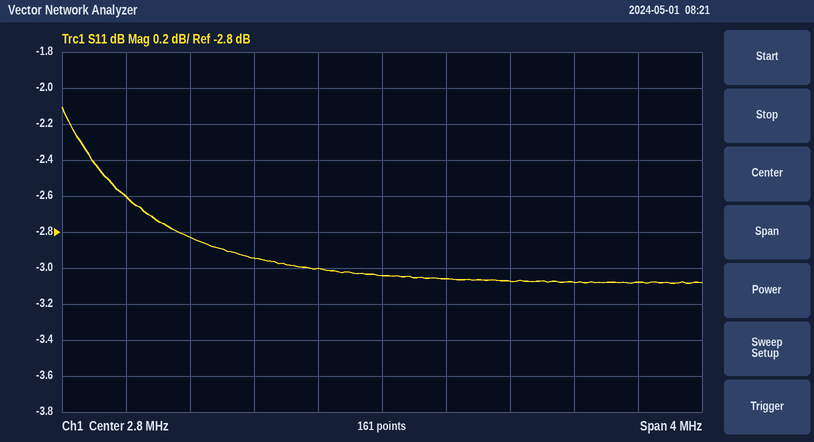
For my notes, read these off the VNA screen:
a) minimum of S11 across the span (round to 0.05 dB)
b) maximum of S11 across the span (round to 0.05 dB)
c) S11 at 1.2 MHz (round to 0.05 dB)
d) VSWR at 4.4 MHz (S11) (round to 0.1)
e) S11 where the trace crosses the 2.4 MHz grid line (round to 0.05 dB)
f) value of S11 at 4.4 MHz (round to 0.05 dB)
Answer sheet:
-3.10 dB
-2.10 dB
-2.60 dB
5.7
-3.00 dB
-3.10 dB
